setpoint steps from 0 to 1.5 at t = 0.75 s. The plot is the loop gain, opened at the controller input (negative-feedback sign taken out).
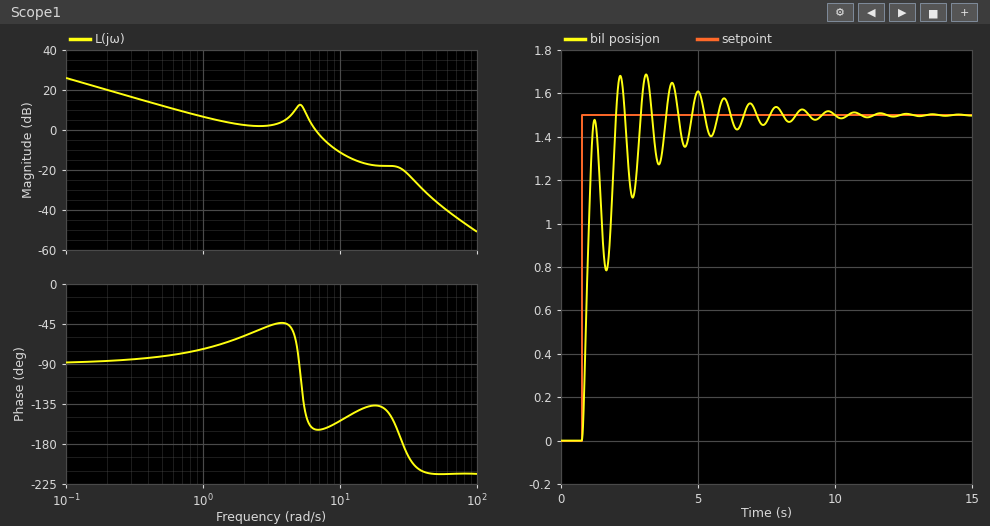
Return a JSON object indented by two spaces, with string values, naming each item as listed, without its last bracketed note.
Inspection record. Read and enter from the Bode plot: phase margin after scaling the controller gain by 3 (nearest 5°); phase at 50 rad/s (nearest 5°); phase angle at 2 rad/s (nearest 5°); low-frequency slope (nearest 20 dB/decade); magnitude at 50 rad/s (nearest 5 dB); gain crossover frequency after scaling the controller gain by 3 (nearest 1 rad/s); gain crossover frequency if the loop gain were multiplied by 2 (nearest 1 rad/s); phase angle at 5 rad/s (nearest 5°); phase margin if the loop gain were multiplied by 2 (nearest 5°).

{
  "phase margin after scaling the controller gain by 3": "25°",
  "phase at 50 rad/s": "-215°",
  "phase angle at 2 rad/s": "-60°",
  "low-frequency slope": "-20 dB/decade",
  "magnitude at 50 rad/s": "-35 dB",
  "gain crossover frequency after scaling the controller gain by 3": "9 rad/s",
  "gain crossover frequency if the loop gain were multiplied by 2": "8 rad/s",
  "phase angle at 5 rad/s": "-85°",
  "phase margin if the loop gain were multiplied by 2": "20°"
}
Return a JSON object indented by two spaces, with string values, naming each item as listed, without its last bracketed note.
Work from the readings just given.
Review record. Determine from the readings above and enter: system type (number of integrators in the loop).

{
  "system type": "1"
}
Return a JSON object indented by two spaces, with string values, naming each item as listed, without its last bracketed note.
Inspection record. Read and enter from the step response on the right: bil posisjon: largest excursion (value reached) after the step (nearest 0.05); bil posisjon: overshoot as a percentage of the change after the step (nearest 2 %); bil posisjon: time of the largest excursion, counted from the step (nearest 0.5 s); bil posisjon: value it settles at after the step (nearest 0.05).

{
  "bil posisjon: largest excursion (value reached) after the step": "1.70",
  "bil posisjon: overshoot as a percentage of the change after the step": "12 %",
  "bil posisjon: time of the largest excursion, counted from the step": "2.5 s",
  "bil posisjon: value it settles at after the step": "1.50"
}
